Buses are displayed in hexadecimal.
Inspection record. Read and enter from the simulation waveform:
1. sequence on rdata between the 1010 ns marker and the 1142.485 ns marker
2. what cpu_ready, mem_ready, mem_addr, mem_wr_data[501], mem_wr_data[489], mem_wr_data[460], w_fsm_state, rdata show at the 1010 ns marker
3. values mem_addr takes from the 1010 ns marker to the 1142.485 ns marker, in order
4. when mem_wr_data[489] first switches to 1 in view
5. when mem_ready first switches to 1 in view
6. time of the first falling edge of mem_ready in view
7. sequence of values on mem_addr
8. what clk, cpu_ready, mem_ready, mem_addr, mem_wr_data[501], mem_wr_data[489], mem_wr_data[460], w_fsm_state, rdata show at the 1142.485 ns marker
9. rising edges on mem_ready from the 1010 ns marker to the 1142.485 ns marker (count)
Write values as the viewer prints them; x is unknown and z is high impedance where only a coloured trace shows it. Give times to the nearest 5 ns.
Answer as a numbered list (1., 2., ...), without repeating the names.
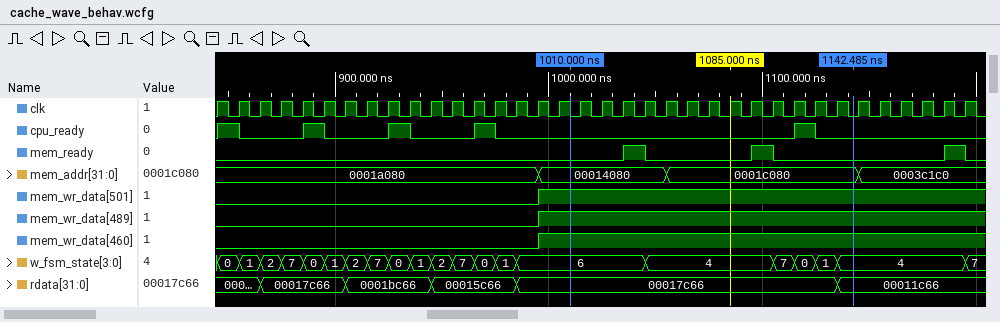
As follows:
1. 00017c66, 00011c66
2. cpu_ready=0, mem_ready=0, mem_addr=00014080, mem_wr_data[501]=1, mem_wr_data[489]=1, mem_wr_data[460]=1, w_fsm_state=6, rdata=00017c66
3. 00014080, 0001c080
4. 995 ns
5. 1035 ns
6. 1045 ns
7. 0001a080, 00014080, 0001c080, 0003c1c0
8. clk=0, cpu_ready=0, mem_ready=0, mem_addr=0001c080, mem_wr_data[501]=1, mem_wr_data[489]=1, mem_wr_data[460]=1, w_fsm_state=4, rdata=00011c66
9. 2
